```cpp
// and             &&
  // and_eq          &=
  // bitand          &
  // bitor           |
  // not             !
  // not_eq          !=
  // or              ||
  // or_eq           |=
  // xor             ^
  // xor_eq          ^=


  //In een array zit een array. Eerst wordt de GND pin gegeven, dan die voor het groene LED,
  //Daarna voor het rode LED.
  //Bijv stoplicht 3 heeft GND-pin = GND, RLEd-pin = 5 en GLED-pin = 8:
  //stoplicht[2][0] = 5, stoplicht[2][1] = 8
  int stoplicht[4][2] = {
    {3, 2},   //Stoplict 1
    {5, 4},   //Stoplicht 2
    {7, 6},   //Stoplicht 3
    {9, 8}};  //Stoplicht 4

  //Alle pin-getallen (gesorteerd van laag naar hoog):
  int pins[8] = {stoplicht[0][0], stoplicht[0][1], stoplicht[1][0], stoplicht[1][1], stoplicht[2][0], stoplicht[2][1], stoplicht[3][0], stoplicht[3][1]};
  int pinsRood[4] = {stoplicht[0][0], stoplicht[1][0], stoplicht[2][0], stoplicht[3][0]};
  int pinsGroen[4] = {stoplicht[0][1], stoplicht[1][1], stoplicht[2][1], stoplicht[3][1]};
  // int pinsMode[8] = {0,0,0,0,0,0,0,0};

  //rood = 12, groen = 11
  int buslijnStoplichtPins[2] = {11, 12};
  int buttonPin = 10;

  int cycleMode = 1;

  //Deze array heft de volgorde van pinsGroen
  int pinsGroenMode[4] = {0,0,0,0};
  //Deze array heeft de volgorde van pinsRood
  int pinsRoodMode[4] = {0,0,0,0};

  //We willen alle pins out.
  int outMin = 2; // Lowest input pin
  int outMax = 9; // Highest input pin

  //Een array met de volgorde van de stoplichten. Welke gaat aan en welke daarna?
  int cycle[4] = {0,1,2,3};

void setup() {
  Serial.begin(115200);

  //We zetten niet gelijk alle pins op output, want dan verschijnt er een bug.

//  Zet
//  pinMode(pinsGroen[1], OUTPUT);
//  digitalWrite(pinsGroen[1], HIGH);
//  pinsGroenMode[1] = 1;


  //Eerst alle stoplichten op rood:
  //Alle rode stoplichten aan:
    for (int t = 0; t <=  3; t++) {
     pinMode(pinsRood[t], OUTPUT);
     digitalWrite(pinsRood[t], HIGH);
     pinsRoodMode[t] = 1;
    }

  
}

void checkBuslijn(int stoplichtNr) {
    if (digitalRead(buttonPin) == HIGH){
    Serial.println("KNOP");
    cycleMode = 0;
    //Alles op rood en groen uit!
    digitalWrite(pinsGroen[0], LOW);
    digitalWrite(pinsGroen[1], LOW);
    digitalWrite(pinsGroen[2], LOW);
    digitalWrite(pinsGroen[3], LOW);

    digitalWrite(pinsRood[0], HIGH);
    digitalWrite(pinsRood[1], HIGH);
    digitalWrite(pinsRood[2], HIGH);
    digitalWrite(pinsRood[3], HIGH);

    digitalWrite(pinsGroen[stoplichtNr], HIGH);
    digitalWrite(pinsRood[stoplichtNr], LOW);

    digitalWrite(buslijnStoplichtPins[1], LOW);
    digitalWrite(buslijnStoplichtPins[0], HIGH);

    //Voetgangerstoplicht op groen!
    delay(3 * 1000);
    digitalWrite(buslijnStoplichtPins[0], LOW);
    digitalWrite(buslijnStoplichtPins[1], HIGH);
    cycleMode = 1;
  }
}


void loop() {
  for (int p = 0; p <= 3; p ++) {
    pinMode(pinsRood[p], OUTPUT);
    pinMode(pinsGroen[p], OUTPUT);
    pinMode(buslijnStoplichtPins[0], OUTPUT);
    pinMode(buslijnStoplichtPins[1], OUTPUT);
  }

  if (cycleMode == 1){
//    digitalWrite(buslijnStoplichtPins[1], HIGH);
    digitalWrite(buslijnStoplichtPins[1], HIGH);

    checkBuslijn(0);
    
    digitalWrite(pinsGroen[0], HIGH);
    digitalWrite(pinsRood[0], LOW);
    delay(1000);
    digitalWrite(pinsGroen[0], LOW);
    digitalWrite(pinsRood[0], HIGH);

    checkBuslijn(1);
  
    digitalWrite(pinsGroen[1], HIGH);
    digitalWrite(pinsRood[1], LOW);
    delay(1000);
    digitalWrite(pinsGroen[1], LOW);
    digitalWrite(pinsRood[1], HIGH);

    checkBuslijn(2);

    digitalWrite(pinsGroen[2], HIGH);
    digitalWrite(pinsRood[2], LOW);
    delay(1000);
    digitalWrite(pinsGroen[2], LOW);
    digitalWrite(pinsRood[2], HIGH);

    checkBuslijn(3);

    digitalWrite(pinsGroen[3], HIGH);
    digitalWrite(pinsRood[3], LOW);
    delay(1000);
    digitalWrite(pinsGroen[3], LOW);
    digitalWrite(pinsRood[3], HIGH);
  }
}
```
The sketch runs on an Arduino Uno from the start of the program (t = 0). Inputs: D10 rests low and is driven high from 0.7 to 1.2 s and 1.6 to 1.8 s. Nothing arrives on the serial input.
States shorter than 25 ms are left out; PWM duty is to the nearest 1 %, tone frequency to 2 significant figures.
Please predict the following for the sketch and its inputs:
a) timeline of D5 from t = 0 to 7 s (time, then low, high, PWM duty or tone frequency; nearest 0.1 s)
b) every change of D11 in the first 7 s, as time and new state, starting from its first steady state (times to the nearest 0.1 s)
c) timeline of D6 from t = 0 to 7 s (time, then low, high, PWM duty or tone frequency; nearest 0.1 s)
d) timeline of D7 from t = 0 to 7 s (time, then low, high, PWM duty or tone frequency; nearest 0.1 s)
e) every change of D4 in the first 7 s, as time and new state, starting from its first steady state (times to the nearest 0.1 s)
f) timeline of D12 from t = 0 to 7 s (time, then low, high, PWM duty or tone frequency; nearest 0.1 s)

0 s high; 1 s low; 5 s high
0 s low; 1 s high; 4 s low
0 s low; 5 s high; 6 s low
0 s high; 5 s low; 6 s high
0 s low; 1 s high; 5 s low
0 s high; 1 s low; 4 s high
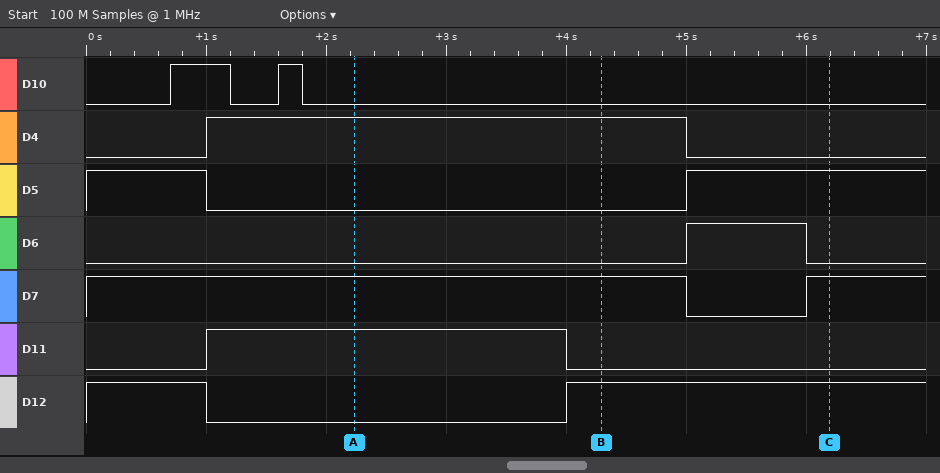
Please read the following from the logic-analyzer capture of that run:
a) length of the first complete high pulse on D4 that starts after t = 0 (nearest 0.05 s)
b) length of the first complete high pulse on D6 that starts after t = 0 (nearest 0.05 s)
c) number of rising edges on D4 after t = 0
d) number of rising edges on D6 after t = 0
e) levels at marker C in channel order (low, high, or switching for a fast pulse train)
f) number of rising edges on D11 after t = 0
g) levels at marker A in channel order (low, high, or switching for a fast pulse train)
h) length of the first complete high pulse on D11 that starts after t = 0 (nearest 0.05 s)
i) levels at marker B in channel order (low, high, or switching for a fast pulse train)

4.00 s
1.00 s
1
1
D10 low, D4 low, D5 high, D6 low, D7 high, D11 low, D12 high
1
D10 low, D4 high, D5 low, D6 low, D7 high, D11 high, D12 low
3.00 s
D10 low, D4 high, D5 low, D6 low, D7 high, D11 low, D12 high
